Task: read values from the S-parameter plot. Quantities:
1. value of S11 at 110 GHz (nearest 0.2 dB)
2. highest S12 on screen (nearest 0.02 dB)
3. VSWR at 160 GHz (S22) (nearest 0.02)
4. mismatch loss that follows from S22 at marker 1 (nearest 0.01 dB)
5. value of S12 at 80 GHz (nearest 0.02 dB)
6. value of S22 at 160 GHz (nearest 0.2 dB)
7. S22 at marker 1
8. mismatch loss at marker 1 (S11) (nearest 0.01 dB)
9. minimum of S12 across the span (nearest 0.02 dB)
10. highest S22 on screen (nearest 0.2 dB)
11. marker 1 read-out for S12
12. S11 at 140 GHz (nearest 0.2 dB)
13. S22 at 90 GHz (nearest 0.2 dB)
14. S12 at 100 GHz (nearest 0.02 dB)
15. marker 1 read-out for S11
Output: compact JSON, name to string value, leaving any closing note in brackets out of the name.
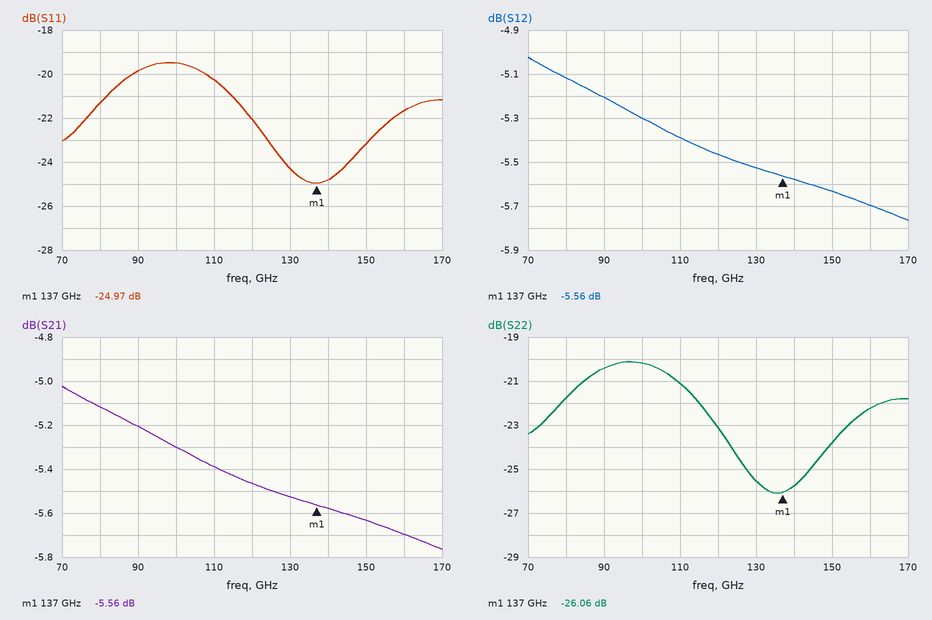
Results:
{"value of S11 at 110 GHz": "-20.2 dB", "highest S12 on screen": "-5.02 dB", "VSWR at 160 GHz (S22)": "1.16", "mismatch loss that follows from S22 at marker 1": "0.01 dB", "value of S12 at 80 GHz": "-5.12 dB", "value of S22 at 160 GHz": "-22.2 dB", "S22 at marker 1": "-26.06 dB", "mismatch loss at marker 1 (S11)": "0.01 dB", "minimum of S12 across the span": "-5.76 dB", "highest S22 on screen": "-20.2 dB", "marker 1 read-out for S12": "-5.56 dB", "S11 at 140 GHz": "-24.8 dB", "S22 at 90 GHz": "-20.4 dB", "S12 at 100 GHz": "-5.30 dB", "marker 1 read-out for S11": "-24.97 dB"}
